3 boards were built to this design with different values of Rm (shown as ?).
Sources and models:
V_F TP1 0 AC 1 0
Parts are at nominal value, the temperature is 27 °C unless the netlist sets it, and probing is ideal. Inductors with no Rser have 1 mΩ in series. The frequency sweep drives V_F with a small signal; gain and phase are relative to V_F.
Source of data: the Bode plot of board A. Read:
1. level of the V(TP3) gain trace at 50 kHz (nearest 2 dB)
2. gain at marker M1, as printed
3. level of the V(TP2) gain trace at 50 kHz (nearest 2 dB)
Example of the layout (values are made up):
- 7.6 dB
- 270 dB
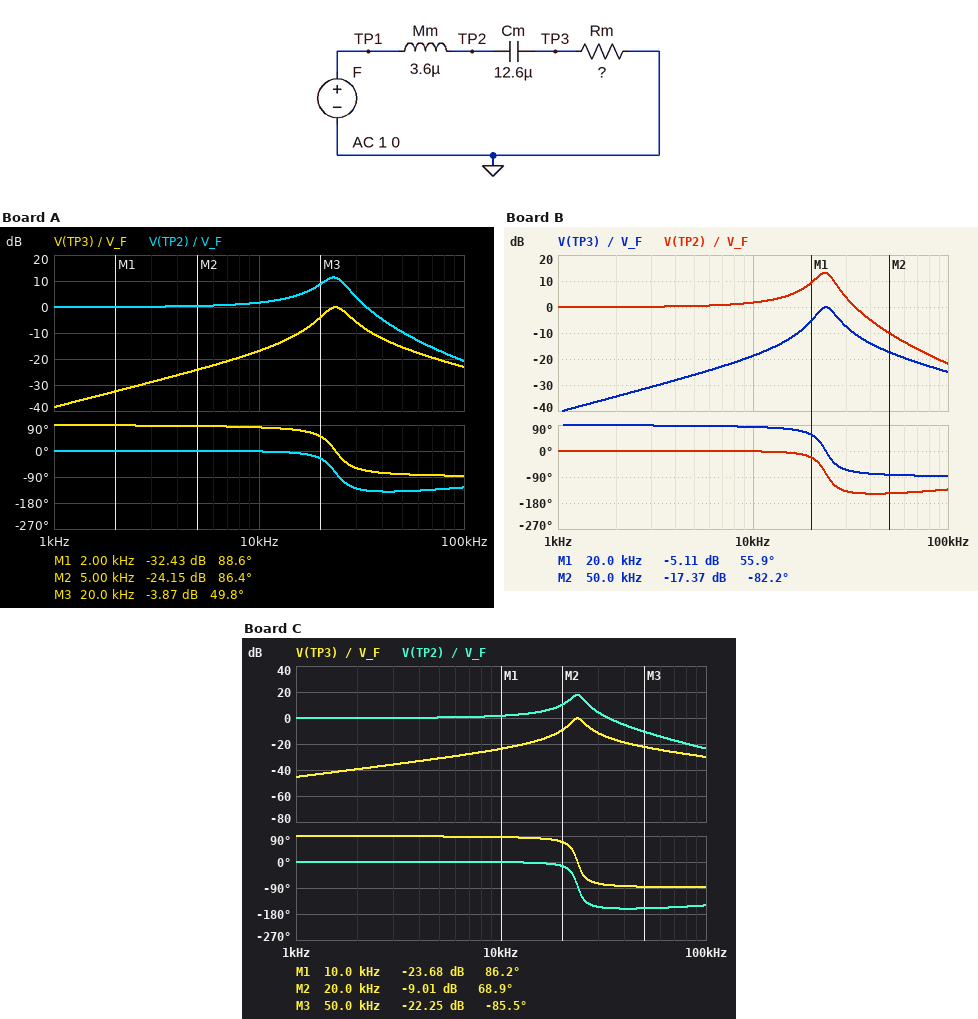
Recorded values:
- -16 dB
- -32.43 dB
- -10 dB
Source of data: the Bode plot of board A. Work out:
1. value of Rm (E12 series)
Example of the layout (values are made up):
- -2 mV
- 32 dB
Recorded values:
- 0.15 Ω
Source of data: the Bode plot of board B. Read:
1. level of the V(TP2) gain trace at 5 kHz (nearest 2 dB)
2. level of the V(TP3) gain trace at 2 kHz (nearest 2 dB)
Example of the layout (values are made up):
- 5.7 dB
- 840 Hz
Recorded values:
- 0 dB
- -34 dB
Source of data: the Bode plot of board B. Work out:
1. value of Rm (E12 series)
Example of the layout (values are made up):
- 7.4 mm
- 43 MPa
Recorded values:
- 0.12 Ω
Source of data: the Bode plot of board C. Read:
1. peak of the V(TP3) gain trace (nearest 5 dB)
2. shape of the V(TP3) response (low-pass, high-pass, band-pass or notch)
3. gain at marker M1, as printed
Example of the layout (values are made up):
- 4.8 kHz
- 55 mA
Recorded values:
- 0 dB
- band-pass
- -23.68 dB
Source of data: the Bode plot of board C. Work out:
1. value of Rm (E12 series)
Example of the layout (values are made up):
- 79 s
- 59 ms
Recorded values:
- 0.068 Ω
